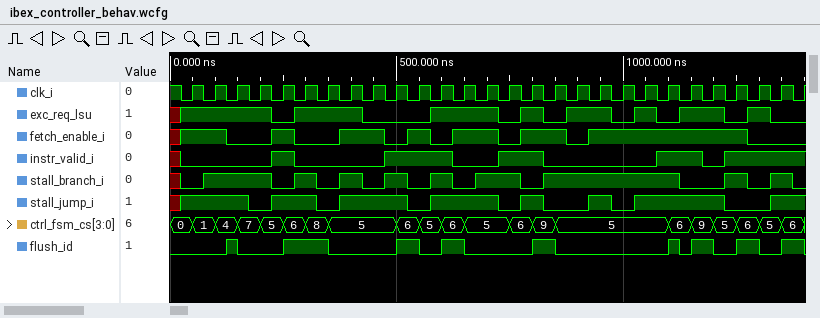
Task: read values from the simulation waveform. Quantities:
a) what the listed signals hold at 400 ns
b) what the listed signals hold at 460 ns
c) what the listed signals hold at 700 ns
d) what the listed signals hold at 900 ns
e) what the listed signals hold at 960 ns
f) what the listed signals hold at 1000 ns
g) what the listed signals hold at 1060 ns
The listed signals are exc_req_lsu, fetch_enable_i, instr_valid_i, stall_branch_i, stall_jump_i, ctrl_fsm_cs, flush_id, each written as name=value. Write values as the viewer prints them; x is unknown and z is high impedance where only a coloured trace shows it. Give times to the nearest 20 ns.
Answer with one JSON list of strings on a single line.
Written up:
["exc_req_lsu=1, fetch_enable_i=1, instr_valid_i=0, stall_branch_i=1, stall_jump_i=1, ctrl_fsm_cs=5, flush_id=0", "exc_req_lsu=0, fetch_enable_i=1, instr_valid_i=0, stall_branch_i=0, stall_jump_i=1, ctrl_fsm_cs=5, flush_id=0", "exc_req_lsu=1, fetch_enable_i=1, instr_valid_i=0, stall_branch_i=1, stall_jump_i=1, ctrl_fsm_cs=5, flush_id=0", "exc_req_lsu=1, fetch_enable_i=0, instr_valid_i=0, stall_branch_i=1, stall_jump_i=0, ctrl_fsm_cs=5, flush_id=0", "exc_req_lsu=1, fetch_enable_i=1, instr_valid_i=0, stall_branch_i=1, stall_jump_i=1, ctrl_fsm_cs=5, flush_id=0", "exc_req_lsu=0, fetch_enable_i=1, instr_valid_i=0, stall_branch_i=1, stall_jump_i=0, ctrl_fsm_cs=5, flush_id=0", "exc_req_lsu=1, fetch_enable_i=1, instr_valid_i=0, stall_branch_i=1, stall_jump_i=1, ctrl_fsm_cs=5, flush_id=0"]
